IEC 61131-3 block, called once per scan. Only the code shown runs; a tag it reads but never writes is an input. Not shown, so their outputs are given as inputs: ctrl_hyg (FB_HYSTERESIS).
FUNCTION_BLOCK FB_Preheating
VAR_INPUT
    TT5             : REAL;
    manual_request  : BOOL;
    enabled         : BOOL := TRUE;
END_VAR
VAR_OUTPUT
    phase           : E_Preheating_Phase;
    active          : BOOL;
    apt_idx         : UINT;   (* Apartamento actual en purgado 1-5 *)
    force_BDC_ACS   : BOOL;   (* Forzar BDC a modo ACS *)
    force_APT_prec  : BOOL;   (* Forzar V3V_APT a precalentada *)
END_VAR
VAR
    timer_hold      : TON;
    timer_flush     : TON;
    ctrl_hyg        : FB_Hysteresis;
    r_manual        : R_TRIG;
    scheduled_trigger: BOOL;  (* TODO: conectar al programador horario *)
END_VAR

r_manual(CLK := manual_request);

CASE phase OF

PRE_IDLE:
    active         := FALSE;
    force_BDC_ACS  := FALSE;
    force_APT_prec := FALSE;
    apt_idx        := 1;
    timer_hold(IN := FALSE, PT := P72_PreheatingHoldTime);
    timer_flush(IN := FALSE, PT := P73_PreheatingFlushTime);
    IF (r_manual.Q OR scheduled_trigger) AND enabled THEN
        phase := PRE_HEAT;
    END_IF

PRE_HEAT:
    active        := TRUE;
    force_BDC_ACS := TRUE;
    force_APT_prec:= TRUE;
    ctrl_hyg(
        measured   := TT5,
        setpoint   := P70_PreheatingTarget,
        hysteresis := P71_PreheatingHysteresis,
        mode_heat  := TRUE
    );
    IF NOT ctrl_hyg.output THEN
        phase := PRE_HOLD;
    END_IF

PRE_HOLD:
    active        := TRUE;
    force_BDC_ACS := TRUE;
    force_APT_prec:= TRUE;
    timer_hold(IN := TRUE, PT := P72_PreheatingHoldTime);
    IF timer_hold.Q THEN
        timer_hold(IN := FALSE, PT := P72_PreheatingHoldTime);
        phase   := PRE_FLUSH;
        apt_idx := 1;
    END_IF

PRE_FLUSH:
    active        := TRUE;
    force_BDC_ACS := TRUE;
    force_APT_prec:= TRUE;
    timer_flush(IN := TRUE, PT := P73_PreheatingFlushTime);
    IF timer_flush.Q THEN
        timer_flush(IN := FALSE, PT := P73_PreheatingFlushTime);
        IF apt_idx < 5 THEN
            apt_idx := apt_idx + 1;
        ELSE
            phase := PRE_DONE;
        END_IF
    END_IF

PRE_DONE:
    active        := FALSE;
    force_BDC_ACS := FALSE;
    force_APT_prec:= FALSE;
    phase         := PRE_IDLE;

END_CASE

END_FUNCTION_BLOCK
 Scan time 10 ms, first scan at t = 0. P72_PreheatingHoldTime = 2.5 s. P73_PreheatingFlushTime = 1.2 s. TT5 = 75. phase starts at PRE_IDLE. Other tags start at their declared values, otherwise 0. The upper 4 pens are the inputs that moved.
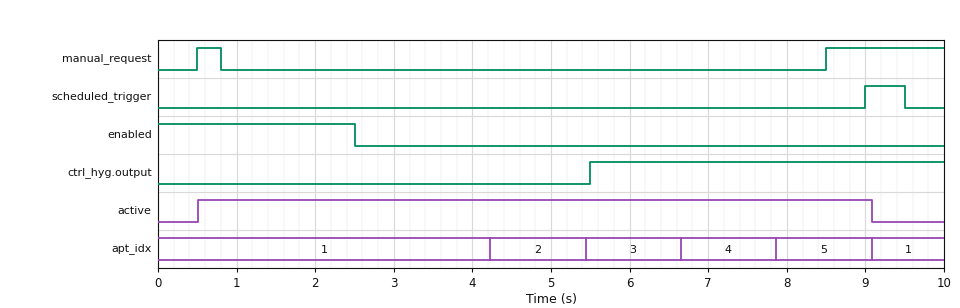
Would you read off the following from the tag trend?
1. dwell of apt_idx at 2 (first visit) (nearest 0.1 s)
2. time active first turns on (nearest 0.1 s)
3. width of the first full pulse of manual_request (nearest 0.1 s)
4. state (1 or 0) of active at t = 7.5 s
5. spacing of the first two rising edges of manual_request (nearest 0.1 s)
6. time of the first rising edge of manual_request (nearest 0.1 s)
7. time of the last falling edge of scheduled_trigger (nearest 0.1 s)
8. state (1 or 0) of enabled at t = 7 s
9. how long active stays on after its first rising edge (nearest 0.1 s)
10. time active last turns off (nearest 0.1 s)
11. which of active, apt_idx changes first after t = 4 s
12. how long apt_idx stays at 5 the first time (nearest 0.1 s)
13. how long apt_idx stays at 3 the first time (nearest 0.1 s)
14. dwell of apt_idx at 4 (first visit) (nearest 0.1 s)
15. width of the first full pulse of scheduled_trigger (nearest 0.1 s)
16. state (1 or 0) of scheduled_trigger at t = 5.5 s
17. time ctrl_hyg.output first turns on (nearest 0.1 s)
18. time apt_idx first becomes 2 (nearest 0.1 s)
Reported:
1.2 s
0.5 s
0.3 s
1
8.0 s
0.5 s
9.5 s
0
8.6 s
9.1 s
apt_idx
1.2 s
1.2 s
1.2 s
0.5 s
0
5.5 s
4.2 s
